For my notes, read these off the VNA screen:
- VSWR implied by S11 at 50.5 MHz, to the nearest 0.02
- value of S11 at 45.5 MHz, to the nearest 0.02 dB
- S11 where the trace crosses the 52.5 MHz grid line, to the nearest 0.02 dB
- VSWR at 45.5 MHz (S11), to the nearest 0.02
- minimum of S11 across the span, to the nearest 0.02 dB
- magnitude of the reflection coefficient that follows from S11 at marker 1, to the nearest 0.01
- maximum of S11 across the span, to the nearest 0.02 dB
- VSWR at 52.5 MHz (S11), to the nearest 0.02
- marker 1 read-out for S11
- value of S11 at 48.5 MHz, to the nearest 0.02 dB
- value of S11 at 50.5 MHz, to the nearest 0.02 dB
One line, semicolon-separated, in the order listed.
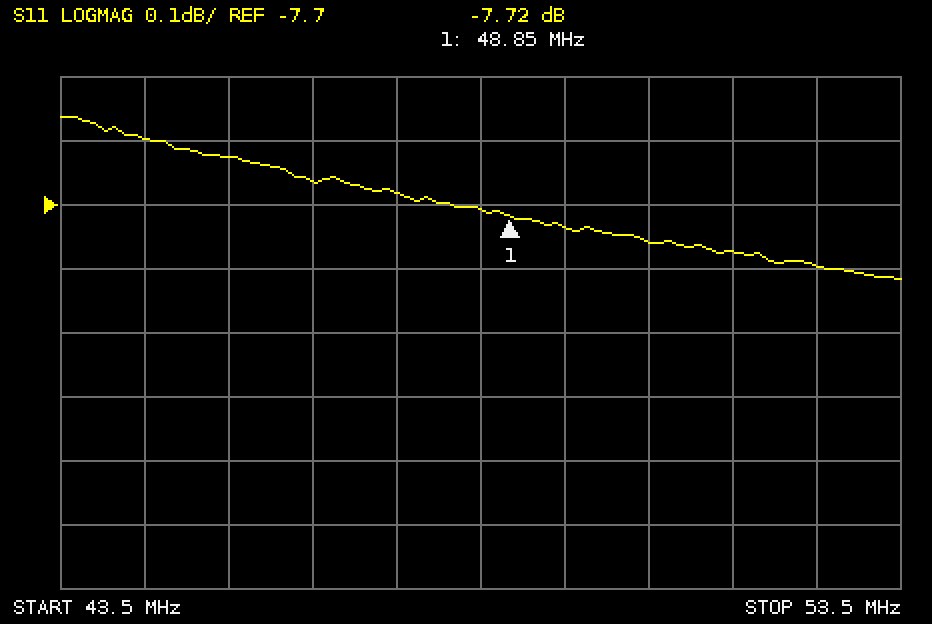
2.38; -7.62 dB; -7.80 dB; 2.42; -7.82 dB; 0.41; -7.56 dB; 2.38; -7.72 dB; -7.70 dB; -7.76 dB
